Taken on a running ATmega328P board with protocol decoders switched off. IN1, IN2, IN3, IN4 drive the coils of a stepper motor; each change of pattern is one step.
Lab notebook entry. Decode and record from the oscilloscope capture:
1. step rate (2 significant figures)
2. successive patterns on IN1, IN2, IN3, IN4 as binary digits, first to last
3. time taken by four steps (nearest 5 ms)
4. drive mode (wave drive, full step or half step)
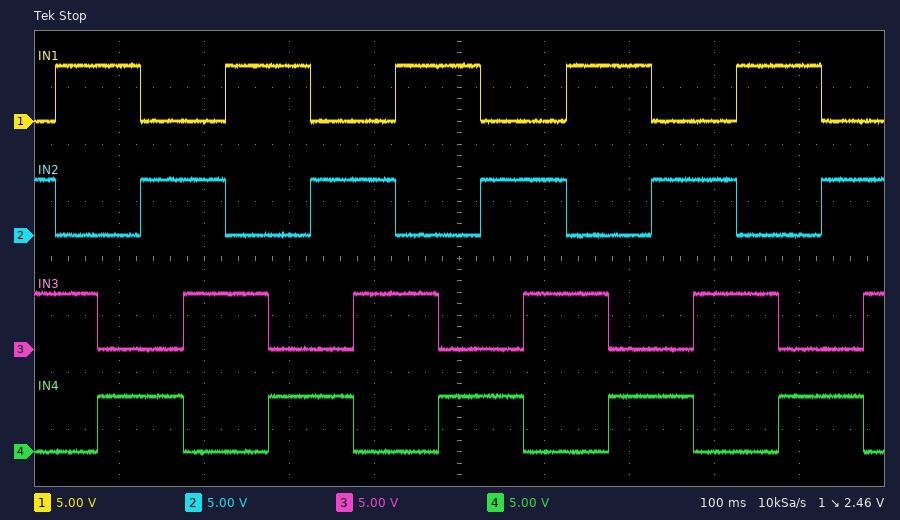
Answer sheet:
20 steps/s
0110 1010 1001 0101 0110 1010 1001 0101 0110 1010 1001 0101 0110 1010 1001 0101 0110 1010 1001 0101 0110
200 ms
full step
